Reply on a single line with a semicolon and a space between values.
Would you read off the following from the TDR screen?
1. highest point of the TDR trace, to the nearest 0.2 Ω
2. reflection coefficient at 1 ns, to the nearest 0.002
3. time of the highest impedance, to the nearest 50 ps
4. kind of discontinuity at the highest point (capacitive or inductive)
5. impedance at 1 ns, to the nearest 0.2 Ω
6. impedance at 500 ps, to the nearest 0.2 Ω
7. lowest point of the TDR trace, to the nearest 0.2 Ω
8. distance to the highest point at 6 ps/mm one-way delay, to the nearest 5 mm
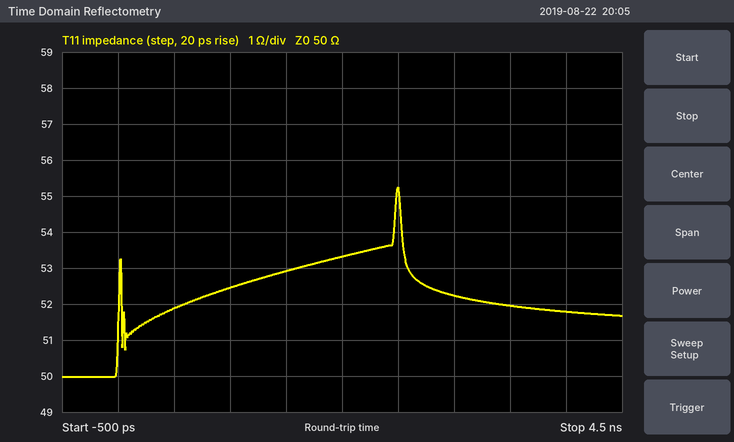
55.2 Ω; +0.024; 2.50 ns; inductive; 52.4 Ω; 51.8 Ω; 50.0 Ω; 210 mm
